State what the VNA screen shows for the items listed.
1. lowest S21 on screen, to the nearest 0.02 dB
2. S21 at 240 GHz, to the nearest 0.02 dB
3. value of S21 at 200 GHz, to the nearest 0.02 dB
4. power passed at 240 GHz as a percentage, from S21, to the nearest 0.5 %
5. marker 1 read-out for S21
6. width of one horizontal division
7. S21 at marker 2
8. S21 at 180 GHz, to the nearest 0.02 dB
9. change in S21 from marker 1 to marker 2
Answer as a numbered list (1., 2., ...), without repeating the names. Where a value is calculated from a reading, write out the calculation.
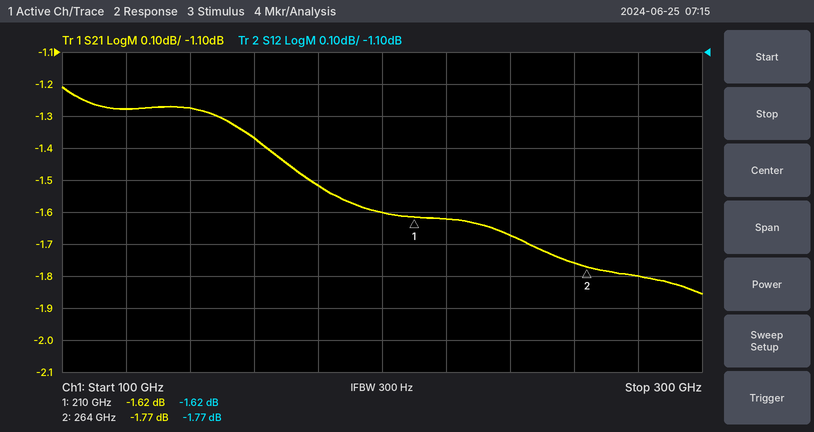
1. -1.86 dB
2. -1.68 dB
3. -1.60 dB
4. 10^(-1.68/10) ≈ 67.9 %, so 68.0 % to the nearest 0.5 %
5. -1.62 dB
6. 20 GHz
7. -1.77 dB
8. -1.52 dB
9. -1.77 − (-1.62) = -0.15 dB
